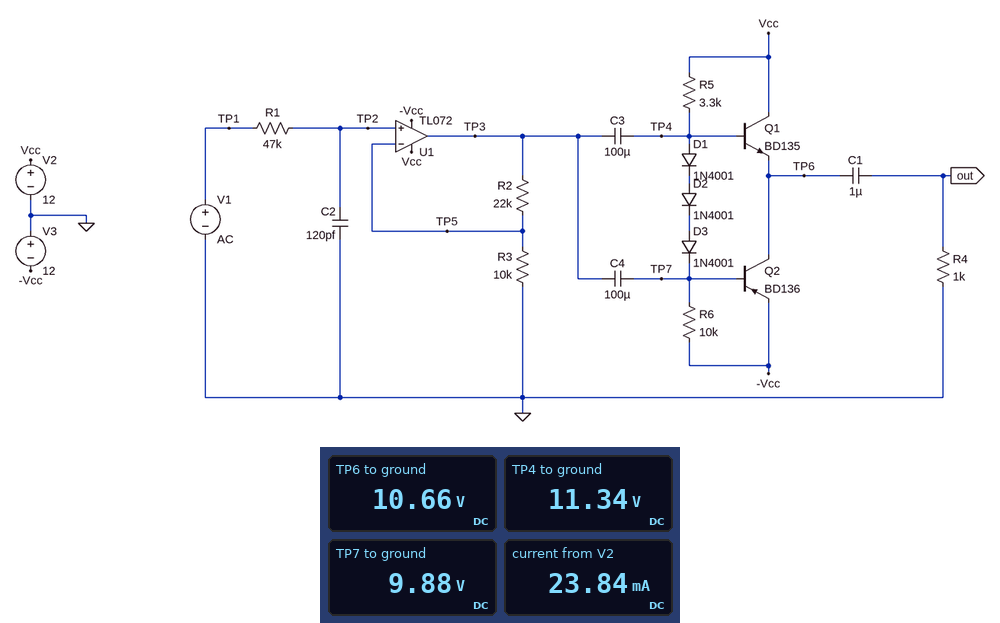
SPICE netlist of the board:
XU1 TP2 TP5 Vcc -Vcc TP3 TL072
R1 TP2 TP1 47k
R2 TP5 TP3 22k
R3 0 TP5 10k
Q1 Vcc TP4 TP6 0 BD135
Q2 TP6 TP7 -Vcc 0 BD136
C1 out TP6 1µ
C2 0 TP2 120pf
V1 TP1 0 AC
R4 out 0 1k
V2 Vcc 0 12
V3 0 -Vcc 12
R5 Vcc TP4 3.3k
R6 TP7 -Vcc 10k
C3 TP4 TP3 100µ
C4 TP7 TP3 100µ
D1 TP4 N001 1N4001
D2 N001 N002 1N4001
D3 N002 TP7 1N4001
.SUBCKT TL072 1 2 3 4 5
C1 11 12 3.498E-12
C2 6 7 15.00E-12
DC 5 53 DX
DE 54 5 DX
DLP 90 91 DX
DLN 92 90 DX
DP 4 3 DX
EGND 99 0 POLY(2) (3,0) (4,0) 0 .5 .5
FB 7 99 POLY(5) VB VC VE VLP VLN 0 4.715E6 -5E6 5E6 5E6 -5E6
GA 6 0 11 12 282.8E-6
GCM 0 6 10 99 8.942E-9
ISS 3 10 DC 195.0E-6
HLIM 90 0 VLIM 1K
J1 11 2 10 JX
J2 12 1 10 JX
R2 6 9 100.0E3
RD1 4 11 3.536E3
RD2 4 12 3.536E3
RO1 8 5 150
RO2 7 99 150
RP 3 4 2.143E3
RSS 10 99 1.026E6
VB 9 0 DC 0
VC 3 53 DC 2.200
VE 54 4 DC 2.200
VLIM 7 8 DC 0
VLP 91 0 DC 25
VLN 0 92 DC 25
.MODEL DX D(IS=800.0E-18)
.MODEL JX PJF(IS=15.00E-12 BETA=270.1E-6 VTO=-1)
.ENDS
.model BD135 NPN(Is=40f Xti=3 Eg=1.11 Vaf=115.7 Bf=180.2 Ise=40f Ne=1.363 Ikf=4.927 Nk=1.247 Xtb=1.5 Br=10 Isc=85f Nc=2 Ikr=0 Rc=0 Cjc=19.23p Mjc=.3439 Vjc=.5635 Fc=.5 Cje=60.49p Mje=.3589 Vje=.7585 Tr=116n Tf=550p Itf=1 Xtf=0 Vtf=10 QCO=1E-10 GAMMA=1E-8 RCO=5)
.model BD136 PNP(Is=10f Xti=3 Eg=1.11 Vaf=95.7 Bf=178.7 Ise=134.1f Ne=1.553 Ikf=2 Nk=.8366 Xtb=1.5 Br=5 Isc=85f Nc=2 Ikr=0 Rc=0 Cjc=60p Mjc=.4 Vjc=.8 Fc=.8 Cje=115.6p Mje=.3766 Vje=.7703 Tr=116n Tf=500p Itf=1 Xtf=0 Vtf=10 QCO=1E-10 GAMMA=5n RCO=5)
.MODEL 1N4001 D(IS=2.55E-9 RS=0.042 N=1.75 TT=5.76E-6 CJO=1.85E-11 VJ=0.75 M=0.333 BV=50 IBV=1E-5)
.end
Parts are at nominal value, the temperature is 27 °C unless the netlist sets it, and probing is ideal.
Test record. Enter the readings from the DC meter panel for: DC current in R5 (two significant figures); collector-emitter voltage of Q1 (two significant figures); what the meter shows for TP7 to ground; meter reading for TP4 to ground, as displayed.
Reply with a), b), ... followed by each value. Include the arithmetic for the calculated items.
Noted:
a) (12 V - 11.34 V) / 3.3 kΩ = 200 µA
b) 12 V - 10.66 V = 1.3 V
c) 9.88 V
d) 11.34 V
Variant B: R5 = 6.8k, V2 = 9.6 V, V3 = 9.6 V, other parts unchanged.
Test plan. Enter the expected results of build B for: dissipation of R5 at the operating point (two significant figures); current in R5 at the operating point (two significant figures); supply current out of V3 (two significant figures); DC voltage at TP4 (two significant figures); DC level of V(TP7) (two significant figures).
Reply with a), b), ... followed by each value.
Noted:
a) 170 µW
b) 160 µA
c) 19 mA
d) 8.5 V
e) 7.1 V
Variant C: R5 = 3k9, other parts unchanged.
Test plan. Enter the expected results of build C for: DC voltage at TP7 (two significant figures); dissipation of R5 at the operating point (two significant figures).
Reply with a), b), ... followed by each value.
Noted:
a) 9.8 V
b) 150 µW
